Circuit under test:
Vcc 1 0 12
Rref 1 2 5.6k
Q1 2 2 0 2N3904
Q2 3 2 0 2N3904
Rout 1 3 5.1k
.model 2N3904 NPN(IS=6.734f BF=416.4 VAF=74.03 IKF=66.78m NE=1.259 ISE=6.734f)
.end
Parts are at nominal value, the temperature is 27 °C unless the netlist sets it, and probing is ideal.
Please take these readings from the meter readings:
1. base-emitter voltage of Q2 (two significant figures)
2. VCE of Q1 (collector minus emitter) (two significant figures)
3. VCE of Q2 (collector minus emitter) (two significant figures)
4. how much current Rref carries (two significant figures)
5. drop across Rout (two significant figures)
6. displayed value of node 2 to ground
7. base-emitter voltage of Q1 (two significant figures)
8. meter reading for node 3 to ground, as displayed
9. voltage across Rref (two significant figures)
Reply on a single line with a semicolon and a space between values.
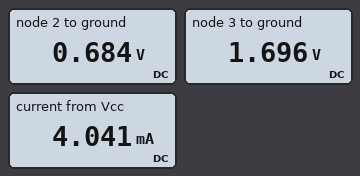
680 mV; 680 mV; 1.7 V; 2.0 mA; 10 V; 0.684 V; 680 mV; 1.696 V; 11 V
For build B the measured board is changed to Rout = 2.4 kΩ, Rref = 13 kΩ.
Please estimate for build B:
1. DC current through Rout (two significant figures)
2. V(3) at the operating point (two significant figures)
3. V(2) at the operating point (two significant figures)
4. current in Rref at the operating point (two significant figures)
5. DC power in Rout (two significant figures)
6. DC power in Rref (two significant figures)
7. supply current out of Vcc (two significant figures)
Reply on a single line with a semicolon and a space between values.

960 µA; 9.7 V; 660 mV; 870 µA; 2.2 mW; 9.9 mW; 1.8 mA
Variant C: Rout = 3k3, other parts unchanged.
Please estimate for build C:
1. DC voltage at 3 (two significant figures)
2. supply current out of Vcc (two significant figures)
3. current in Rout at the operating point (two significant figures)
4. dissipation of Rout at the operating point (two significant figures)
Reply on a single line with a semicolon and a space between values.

5.0 V; 4.1 mA; 2.1 mA; 15 mW
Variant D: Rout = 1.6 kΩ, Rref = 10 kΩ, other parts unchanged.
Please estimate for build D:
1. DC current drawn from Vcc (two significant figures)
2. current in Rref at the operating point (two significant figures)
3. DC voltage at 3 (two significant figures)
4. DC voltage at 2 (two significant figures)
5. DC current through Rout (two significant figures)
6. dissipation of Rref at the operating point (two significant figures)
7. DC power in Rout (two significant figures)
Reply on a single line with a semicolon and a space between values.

2.4 mA; 1.1 mA; 10 V; 670 mV; 1.3 mA; 13 mW; 2.5 mW
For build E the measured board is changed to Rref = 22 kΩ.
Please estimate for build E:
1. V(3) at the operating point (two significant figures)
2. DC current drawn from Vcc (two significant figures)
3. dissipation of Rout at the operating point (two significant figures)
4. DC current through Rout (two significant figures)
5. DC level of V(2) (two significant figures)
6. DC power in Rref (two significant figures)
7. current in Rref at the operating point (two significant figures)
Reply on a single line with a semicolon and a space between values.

9.1 V; 1.1 mA; 1.6 mW; 570 µA; 650 mV; 5.9 mW; 520 µA
